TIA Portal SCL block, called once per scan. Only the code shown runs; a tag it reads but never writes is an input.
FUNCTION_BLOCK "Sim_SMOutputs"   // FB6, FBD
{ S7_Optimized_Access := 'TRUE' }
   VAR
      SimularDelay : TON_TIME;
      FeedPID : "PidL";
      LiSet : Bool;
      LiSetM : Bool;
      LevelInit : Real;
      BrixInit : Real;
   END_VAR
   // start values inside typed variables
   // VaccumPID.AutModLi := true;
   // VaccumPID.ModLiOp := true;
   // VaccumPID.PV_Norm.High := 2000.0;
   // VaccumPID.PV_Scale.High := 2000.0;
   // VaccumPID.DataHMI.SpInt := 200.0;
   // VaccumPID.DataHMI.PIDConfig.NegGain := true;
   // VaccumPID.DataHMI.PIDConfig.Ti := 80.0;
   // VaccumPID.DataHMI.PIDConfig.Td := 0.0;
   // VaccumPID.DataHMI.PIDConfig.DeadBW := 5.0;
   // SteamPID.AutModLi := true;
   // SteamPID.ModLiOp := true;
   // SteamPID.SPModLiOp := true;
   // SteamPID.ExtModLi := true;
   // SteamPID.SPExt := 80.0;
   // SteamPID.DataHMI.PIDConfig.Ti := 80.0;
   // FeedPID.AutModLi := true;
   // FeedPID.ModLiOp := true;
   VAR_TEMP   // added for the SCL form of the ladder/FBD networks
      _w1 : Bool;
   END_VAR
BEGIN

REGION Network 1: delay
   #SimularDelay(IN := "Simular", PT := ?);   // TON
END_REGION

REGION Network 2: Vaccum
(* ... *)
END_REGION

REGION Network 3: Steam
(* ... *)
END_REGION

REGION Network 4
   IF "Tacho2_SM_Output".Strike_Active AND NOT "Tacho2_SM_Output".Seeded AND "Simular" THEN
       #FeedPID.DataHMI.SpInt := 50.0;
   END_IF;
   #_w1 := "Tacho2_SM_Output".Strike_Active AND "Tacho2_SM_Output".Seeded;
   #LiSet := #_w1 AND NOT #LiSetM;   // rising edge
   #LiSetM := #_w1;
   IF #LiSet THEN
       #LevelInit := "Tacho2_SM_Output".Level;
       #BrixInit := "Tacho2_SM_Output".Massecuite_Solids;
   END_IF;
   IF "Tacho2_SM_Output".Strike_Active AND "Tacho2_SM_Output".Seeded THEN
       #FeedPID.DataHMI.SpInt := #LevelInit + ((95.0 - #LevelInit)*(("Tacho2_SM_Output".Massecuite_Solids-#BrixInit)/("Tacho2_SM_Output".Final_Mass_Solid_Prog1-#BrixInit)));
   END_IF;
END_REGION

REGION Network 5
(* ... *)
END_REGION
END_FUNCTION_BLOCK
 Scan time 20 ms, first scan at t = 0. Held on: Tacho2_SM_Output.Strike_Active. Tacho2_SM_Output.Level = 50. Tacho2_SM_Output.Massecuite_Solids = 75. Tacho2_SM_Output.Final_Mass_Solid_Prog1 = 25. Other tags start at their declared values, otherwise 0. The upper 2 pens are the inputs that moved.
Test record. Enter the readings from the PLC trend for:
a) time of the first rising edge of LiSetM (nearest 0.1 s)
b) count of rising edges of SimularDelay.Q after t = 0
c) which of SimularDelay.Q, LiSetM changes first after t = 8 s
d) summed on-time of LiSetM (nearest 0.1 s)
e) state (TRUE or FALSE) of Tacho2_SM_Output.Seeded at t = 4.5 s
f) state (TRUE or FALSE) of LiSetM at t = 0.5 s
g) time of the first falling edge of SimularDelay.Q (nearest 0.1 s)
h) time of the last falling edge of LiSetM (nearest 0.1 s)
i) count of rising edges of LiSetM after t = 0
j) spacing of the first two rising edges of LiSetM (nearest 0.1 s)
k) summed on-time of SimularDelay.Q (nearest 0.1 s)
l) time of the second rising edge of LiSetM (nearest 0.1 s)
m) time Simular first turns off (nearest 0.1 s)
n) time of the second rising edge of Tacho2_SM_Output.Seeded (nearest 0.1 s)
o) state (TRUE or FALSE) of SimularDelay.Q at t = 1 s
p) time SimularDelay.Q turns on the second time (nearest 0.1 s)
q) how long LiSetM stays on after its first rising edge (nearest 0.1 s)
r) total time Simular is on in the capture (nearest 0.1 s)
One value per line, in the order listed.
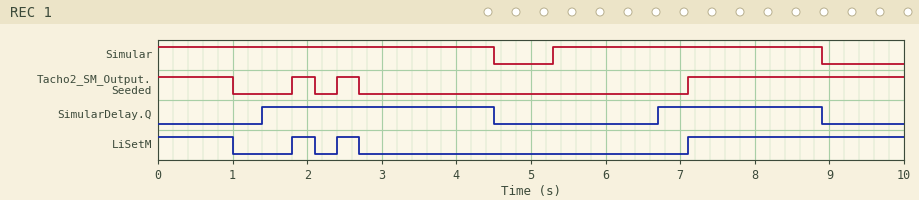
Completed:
1.8 s
2
SimularDelay.Q
4.5 s
FALSE
TRUE
4.5 s
2.7 s
3
0.6 s
5.3 s
2.4 s
4.5 s
2.4 s
FALSE
6.7 s
0.3 s
8.1 s
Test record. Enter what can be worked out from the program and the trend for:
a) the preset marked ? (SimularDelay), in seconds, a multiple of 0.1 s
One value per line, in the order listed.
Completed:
1.4 s
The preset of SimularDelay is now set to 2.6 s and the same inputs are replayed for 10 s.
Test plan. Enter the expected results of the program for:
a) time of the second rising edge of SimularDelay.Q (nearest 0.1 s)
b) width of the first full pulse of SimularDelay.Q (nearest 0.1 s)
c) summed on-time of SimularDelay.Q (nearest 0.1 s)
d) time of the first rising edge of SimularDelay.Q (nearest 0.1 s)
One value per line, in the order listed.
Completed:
7.9 s
1.9 s
2.9 s
2.6 s
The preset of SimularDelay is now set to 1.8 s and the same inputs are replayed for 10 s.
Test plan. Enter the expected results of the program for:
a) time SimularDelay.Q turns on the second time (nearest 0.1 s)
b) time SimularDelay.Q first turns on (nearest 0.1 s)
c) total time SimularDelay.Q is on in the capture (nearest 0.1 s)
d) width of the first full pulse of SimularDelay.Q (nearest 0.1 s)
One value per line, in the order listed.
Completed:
7.1 s
1.8 s
4.5 s
2.7 s
